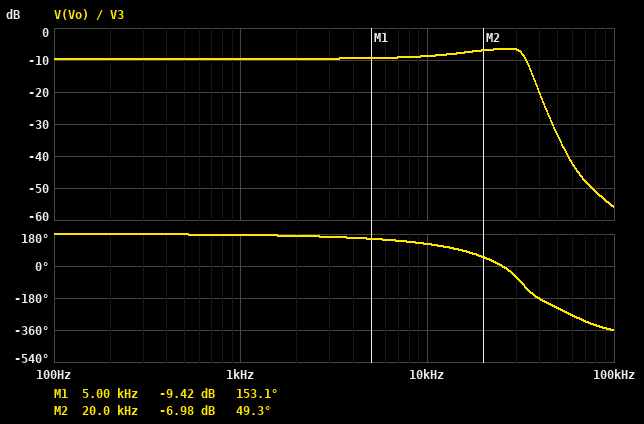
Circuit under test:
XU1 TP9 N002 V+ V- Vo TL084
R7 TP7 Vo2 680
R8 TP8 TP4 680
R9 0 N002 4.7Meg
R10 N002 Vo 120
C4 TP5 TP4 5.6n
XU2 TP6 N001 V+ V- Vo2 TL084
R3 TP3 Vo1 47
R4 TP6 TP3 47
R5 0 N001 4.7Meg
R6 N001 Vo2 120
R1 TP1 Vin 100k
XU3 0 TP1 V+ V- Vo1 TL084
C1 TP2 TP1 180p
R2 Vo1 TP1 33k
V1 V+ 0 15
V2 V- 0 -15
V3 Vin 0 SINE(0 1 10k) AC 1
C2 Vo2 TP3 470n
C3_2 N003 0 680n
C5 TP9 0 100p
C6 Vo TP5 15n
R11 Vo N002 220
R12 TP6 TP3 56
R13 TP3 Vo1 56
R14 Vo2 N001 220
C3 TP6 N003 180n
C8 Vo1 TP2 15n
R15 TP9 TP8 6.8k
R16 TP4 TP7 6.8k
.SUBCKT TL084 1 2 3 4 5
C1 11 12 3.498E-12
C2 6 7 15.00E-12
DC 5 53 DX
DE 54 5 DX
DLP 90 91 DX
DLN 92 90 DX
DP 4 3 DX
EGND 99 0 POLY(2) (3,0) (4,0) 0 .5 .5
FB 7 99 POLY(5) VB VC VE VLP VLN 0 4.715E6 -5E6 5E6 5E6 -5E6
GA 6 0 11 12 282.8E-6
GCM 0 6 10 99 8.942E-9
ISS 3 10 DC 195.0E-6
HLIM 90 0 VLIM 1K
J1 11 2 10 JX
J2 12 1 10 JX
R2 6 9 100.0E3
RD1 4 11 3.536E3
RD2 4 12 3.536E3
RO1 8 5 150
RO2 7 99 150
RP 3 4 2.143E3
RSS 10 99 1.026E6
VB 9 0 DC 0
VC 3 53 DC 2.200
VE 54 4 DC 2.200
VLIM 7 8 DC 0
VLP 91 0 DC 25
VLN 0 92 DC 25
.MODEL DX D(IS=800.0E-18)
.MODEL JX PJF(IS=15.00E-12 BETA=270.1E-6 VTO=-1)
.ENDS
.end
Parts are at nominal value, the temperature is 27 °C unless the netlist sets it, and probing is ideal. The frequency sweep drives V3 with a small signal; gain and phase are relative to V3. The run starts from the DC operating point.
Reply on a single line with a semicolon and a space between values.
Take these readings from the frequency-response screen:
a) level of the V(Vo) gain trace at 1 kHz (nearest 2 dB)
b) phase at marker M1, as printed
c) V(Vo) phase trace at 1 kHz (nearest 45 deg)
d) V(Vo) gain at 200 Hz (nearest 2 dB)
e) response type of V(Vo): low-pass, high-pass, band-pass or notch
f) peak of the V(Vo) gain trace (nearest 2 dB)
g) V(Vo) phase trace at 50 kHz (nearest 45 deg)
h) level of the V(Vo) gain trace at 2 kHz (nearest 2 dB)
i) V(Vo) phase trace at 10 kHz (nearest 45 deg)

-10 dB; 153.1 deg; 180 deg; -10 dB; low-pass; -6 dB; -225 deg; -10 dB; 135 deg
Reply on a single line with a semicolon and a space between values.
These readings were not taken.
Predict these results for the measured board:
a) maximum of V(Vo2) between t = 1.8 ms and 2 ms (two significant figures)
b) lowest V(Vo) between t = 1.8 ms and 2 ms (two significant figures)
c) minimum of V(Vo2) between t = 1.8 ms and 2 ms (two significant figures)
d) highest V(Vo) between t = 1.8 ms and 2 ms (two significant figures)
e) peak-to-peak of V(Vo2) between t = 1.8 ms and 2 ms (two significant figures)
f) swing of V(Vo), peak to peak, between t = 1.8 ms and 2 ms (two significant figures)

330 mV; -360 mV; -330 mV; 360 mV; 660 mV; 730 mV
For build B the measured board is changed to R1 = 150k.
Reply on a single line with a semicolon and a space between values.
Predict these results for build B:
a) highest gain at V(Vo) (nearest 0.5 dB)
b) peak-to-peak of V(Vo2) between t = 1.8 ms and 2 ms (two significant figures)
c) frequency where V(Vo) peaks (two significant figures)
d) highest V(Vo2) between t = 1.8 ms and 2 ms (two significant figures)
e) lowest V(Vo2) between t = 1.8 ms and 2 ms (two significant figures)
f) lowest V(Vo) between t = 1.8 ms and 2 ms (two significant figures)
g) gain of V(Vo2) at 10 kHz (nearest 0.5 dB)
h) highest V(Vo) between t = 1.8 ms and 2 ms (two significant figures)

-10.0 dB; 440 mV; 28 kHz; 220 mV; -220 mV; -240 mV; -13.0 dB; 240 mV
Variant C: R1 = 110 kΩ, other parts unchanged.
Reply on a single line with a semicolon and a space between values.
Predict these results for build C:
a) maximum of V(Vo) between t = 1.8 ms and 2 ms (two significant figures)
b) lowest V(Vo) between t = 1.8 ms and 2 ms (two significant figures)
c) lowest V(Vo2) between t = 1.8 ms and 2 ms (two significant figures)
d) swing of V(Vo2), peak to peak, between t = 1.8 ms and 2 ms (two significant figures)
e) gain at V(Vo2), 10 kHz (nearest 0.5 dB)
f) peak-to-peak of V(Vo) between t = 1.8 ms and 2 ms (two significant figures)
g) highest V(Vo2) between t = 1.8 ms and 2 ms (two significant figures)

330 mV; -330 mV; -300 mV; 600 mV; -10.5 dB; 660 mV; 300 mV
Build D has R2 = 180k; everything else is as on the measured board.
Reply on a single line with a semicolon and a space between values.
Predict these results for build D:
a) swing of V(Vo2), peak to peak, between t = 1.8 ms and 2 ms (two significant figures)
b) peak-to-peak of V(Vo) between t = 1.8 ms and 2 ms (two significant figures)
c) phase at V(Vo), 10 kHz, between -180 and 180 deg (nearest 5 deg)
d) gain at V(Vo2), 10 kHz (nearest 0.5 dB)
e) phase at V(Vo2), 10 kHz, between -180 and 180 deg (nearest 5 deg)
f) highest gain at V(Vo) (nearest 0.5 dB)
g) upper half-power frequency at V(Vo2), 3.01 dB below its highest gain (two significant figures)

1.7 V; 1.9 V; 80 deg; -1.5 dB; 85 deg; 5.0 dB; 5.2 kHz
